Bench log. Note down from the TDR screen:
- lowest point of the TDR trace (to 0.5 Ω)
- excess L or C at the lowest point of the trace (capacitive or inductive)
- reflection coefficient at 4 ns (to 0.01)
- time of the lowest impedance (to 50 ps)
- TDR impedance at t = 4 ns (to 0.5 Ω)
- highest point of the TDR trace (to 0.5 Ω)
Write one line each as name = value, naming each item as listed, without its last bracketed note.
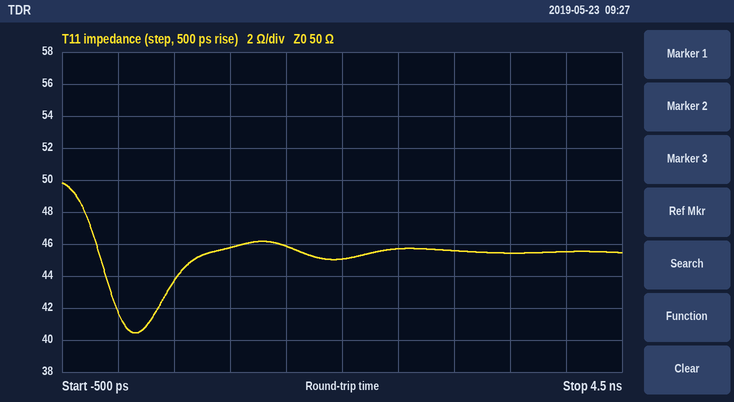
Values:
lowest point of the TDR trace = 40.5 Ω
excess L or C at the lowest point of the trace = capacitive
reflection coefficient at 4 ns = -0.05
time of the lowest impedance = 150 ps
TDR impedance at t = 4 ns = 45.5 Ω
highest point of the TDR trace = 50.0 Ω
